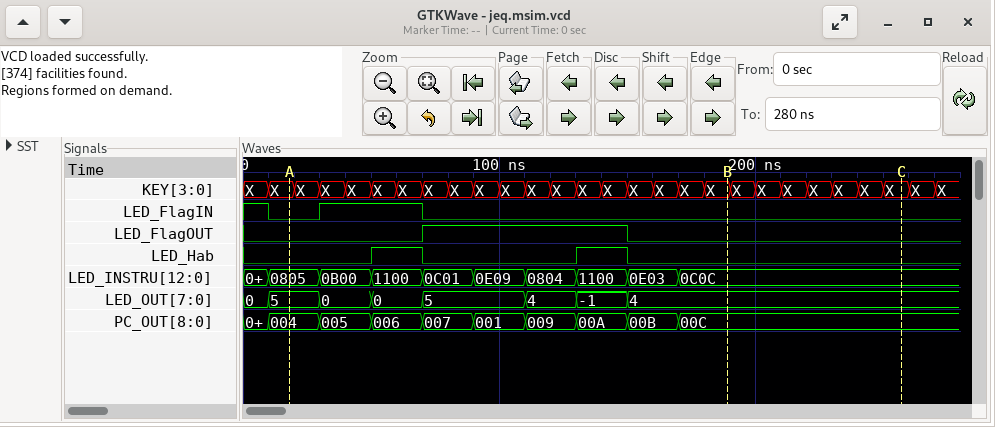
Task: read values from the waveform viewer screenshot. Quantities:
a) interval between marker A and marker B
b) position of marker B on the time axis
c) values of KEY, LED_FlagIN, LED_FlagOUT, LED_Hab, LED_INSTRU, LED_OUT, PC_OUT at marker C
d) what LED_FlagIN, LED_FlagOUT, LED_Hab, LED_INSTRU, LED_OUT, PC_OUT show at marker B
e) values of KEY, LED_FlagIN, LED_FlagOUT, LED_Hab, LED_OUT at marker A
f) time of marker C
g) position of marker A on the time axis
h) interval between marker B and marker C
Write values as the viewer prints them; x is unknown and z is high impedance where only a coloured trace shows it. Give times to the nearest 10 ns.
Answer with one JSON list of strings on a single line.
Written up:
["170 ns", "190 ns", "KEY=X, LED_FlagIN=0, LED_FlagOUT=0, LED_Hab=0, LED_INSTRU=0C0C, LED_OUT=4, PC_OUT=00C", "LED_FlagIN=0, LED_FlagOUT=0, LED_Hab=0, LED_INSTRU=0C0C, LED_OUT=4, PC_OUT=00C", "KEY=X, LED_FlagIN=0, LED_FlagOUT=0, LED_Hab=0, LED_OUT=5", "260 ns", "20 ns", "70 ns"]
